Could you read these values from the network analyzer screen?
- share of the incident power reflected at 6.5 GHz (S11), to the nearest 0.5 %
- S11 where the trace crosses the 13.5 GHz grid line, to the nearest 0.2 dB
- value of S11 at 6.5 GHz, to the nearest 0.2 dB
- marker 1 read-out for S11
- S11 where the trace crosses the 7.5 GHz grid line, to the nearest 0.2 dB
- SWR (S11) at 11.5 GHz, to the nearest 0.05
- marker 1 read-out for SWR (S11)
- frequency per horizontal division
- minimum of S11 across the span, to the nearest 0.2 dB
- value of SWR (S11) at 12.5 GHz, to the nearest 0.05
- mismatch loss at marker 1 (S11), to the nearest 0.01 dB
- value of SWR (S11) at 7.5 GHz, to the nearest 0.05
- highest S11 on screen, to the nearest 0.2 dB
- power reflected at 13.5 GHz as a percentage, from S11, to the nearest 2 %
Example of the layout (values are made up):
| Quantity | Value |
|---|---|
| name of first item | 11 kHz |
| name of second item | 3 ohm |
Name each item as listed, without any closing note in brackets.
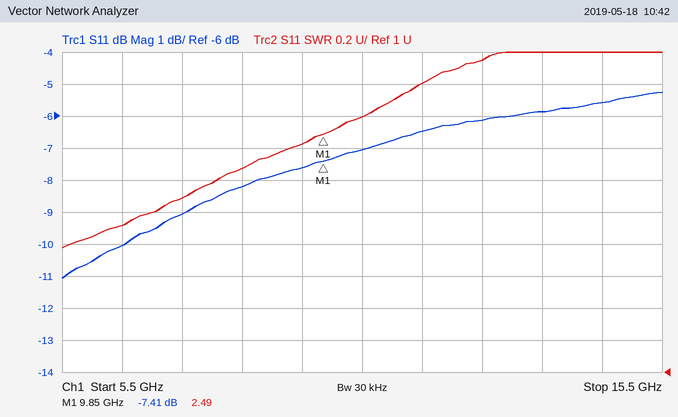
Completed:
| Quantity | Value |
|---|---|
| share of the incident power reflected at 6.5 GHz (S11), to the nearest 0.5 % | 10.0 % |
| S11 where the trace crosses the 13.5 GHz grid line, to the nearest 0.2 dB | -5.8 dB |
| value of S11 at 6.5 GHz, to the nearest 0.2 dB | -10.0 dB |
| marker 1 read-out for S11 | -7.41 dB |
| S11 where the trace crosses the 7.5 GHz grid line, to the nearest 0.2 dB | -9.0 dB |
| SWR (S11) at 11.5 GHz, to the nearest 0.05 | 2.80 |
| marker 1 read-out for SWR | 2.49 |
| frequency per horizontal division | 1 GHz |
| minimum of S11 across the span, to the nearest 0.2 dB | -11.0 dB |
| value of SWR (S11) at 12.5 GHz, to the nearest 0.05 | 2.95 |
| mismatch loss at marker 1 (S11), to the nearest 0.01 dB | 0.87 dB |
| value of SWR (S11) at 7.5 GHz, to the nearest 0.05 | 2.10 |
| highest S11 on screen, to the nearest 0.2 dB | -5.2 dB |
| power reflected at 13.5 GHz as a percentage, from S11, to the nearest 2 % | 26 % |
